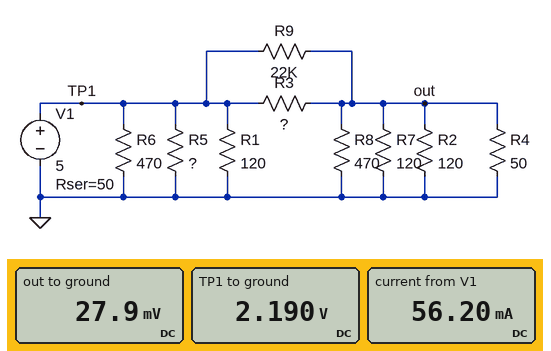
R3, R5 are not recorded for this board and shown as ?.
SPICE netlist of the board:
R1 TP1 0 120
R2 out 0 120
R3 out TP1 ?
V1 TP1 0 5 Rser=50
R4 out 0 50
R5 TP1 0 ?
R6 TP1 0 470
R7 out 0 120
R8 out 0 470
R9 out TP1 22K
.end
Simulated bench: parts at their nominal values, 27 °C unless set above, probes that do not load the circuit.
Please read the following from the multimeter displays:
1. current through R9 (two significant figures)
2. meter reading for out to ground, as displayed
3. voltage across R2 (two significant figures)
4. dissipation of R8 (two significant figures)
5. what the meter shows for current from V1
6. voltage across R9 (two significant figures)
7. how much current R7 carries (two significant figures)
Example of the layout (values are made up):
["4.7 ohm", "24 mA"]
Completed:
["98 µA", "27.9 mV", "28 mV", "1.7 µW", "56.20 mA", "2.2 V", "230 µA"]
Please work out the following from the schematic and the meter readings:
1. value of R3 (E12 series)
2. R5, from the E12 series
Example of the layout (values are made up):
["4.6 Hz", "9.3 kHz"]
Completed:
["2.2 kΩ", "68 Ω"]
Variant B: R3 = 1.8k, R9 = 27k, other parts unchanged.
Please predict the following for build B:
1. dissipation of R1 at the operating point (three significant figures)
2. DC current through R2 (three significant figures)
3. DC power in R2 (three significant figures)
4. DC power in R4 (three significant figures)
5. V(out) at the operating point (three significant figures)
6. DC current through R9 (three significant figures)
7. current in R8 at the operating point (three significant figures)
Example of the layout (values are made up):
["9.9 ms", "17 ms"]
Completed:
["39.8 mW", "274 µA", "9.01 µW", "21.6 µW", "32.9 mV", "79.7 µA", "70.0 µA"]
